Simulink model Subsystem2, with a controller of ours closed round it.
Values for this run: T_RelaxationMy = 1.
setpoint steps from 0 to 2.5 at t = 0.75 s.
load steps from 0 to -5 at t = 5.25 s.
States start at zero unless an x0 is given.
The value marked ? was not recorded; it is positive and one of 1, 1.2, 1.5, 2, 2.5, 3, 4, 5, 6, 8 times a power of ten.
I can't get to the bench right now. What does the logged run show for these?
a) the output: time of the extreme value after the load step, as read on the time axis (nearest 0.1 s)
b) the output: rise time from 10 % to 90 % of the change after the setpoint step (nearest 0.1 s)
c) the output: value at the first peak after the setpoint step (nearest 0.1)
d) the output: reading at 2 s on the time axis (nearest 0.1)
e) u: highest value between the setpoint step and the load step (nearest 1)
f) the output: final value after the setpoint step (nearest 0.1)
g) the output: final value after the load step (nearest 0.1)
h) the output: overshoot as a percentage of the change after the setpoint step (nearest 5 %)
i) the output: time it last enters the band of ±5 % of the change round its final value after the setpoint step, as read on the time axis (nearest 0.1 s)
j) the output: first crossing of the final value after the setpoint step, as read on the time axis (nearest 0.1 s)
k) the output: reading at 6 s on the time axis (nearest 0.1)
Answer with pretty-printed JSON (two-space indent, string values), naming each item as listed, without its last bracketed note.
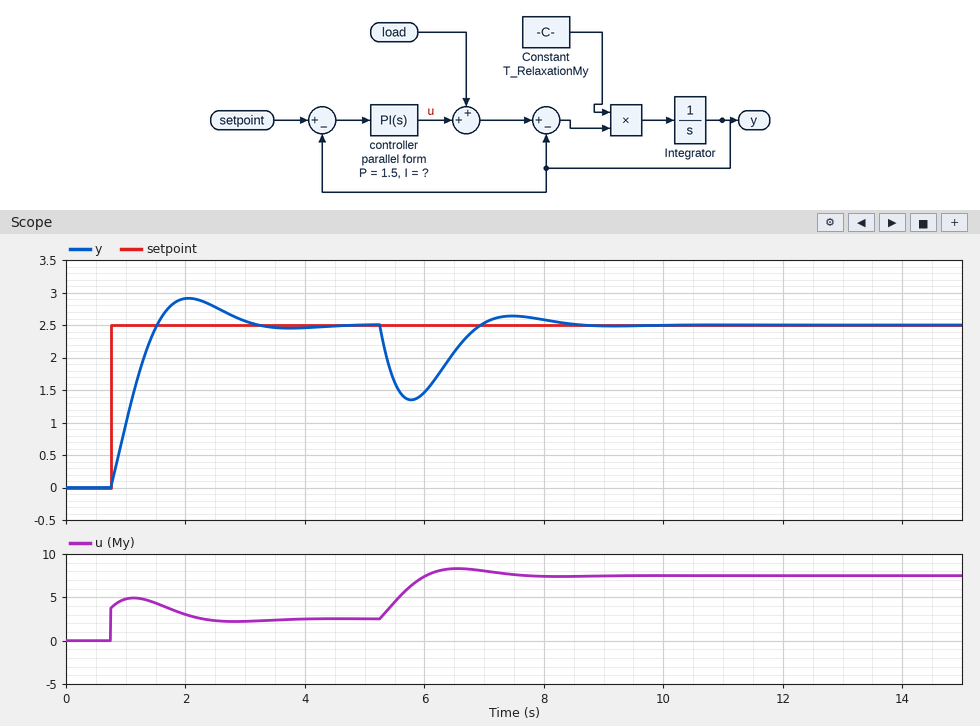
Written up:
{
  "the output: time of the extreme value after the load step, as read on the time axis": "5.8 s",
  "the output: rise time from 10 % to 90 % of the change after the setpoint step": "0.6 s",
  "the output: value at the first peak after the setpoint step": "2.9",
  "the output: reading at 2 s on the time axis": "2.9",
  "u: highest value between the setpoint step and the load step": "5",
  "the output: final value after the setpoint step": "2.5",
  "the output: final value after the load step": "2.5",
  "the output: overshoot as a percentage of the change after the setpoint step": "15 %",
  "the output: time it last enters the band of ±5 % of the change round its final value after the setpoint step, as read on the time axis": "2.8 s",
  "the output: first crossing of the final value after the setpoint step, as read on the time axis": "1.5 s",
  "the output: reading at 6 s on the time axis": "1.5"
}
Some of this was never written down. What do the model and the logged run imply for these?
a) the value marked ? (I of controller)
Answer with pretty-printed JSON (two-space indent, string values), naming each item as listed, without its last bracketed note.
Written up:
{
  "the value marked ?": "5"
}
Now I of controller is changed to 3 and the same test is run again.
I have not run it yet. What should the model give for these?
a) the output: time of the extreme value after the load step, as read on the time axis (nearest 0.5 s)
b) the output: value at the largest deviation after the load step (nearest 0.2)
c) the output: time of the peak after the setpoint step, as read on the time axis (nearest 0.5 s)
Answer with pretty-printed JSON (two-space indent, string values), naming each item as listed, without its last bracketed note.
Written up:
{
  "the output: time of the extreme value after the load step, as read on the time axis": "6.0 s",
  "the output: value at the largest deviation after the load step": "1.2",
  "the output: time of the peak after the setpoint step, as read on the time axis": "2.5 s"
}
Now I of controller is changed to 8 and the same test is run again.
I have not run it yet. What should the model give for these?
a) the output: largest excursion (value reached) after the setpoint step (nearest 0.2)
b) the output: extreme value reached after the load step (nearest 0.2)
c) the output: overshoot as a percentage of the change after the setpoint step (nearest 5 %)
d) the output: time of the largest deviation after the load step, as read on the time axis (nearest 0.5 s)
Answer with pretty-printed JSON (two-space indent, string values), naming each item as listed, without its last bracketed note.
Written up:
{
  "the output: largest excursion (value reached) after the setpoint step": "3.2",
  "the output: extreme value reached after the load step": "1.4",
  "the output: overshoot as a percentage of the change after the setpoint step": "25 %",
  "the output: time of the largest deviation after the load step, as read on the time axis": "5.5 s"
}
